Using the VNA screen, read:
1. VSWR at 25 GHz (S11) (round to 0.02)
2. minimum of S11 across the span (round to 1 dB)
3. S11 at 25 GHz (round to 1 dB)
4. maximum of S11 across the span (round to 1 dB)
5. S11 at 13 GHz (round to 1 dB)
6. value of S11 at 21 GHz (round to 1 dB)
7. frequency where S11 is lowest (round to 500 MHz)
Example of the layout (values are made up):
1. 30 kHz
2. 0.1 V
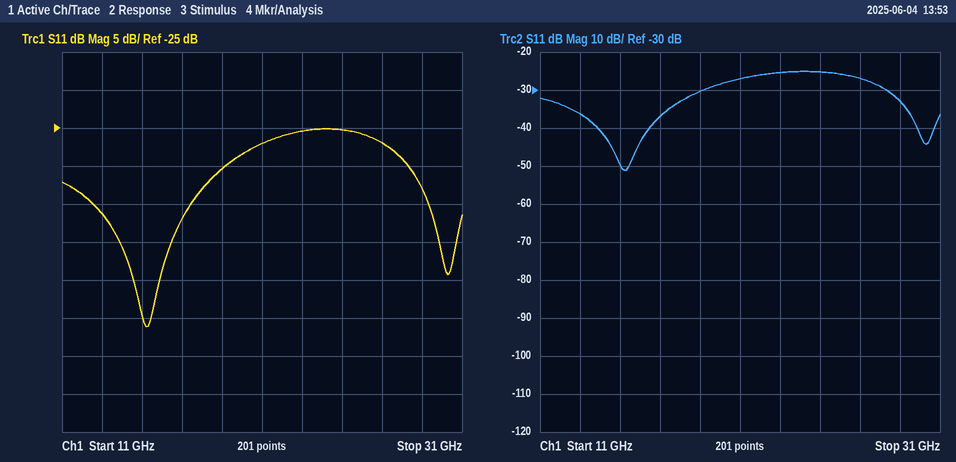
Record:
1. 1.12
2. -51 dB
3. -25 dB
4. -25 dB
5. -36 dB
6. -27 dB
7. 15.0 GHz
